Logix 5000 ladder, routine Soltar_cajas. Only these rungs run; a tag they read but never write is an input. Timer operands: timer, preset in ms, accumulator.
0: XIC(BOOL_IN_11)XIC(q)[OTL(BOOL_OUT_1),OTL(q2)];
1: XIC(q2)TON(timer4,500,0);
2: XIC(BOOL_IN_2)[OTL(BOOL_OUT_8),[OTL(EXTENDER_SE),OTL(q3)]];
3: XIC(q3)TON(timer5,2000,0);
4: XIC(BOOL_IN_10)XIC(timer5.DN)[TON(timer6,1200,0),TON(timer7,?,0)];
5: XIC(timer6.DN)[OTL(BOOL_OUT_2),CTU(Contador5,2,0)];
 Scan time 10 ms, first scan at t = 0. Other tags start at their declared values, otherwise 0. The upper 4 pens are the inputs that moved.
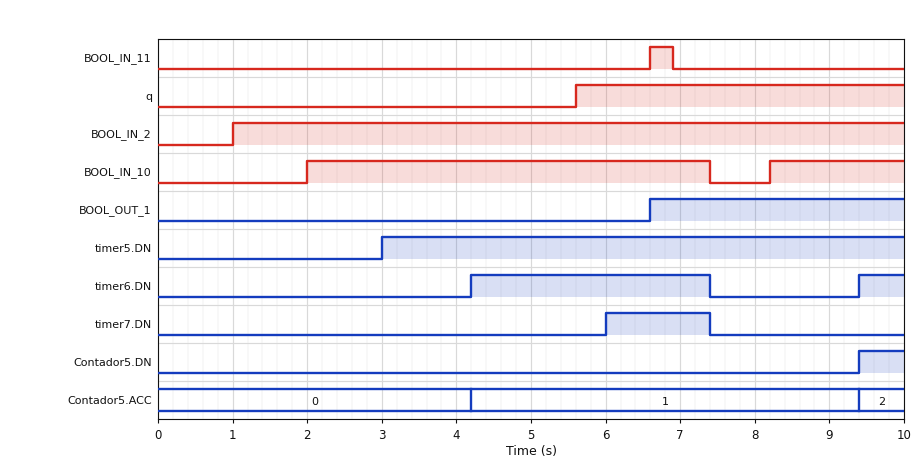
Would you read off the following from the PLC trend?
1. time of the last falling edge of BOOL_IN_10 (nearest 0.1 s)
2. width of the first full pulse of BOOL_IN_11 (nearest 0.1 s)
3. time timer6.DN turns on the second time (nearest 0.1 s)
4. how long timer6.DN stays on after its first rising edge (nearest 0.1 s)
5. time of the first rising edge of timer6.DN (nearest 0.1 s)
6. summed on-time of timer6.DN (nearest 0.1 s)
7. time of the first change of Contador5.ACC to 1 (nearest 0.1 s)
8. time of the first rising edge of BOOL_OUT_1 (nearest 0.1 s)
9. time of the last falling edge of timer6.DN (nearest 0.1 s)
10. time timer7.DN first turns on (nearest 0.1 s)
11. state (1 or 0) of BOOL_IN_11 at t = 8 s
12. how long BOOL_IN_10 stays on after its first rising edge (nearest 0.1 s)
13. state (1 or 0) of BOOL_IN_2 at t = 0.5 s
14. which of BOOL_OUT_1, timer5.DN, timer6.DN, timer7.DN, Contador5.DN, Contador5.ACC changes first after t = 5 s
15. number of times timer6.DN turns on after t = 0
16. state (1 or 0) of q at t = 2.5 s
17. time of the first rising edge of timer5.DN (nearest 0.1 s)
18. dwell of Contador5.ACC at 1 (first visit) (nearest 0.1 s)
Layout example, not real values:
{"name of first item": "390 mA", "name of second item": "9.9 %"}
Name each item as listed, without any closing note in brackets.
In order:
{"time of the last falling edge of BOOL_IN_10": "7.4 s", "width of the first full pulse of BOOL_IN_11": "0.3 s", "time timer6.DN turns on the second time": "9.4 s", "how long timer6.DN stays on after its first rising edge": "3.2 s", "time of the first rising edge of timer6.DN": "4.2 s", "summed on-time of timer6.DN": "3.8 s", "time of the first change of Contador5.ACC to 1": "4.2 s", "time of the first rising edge of BOOL_OUT_1": "6.6 s", "time of the last falling edge of timer6.DN": "7.4 s", "time timer7.DN first turns on": "6.0 s", "state (1 or 0) of BOOL_IN_11 at t = 8 s": "0", "how long BOOL_IN_10 stays on after its first rising edge": "5.4 s", "state (1 or 0) of BOOL_IN_2 at t = 0.5 s": "0", "which of BOOL_OUT_1, timer5.DN, timer6.DN, timer7.DN, Contador5.DN, Contador5.ACC changes first after t = 5 s": "timer7.DN", "number of times timer6.DN turns on after t = 0": "2", "state (1 or 0) of q at t = 2.5 s": "0", "time of the first rising edge of timer5.DN": "3.0 s", "dwell of Contador5.ACC at 1 (first visit)": "5.2 s"}
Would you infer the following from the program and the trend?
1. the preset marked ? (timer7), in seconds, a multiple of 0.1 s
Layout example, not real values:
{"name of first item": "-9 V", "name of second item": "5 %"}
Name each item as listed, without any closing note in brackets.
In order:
{"the preset marked ? (timer7), in seconds, a multiple of 0.1 s": "3.0 s"}
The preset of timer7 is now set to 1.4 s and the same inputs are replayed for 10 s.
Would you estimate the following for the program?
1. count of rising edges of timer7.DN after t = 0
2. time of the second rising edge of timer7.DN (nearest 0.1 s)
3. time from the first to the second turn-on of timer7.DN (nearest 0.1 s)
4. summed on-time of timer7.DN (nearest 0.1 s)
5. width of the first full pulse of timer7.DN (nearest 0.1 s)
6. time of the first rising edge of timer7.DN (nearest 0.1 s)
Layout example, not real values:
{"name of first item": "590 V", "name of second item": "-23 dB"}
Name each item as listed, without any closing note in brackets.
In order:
{"count of rising edges of timer7.DN after t = 0": "2", "time of the second rising edge of timer7.DN": "9.6 s", "time from the first to the second turn-on of timer7.DN": "5.2 s", "summed on-time of timer7.DN": "3.4 s", "width of the first full pulse of timer7.DN": "3.0 s", "time of the first rising edge of timer7.DN": "4.4 s"}
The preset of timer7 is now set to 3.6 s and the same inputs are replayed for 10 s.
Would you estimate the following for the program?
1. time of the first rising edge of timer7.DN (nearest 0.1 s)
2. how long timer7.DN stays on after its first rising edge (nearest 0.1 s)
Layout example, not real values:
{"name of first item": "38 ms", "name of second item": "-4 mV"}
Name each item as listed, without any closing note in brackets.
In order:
{"time of the first rising edge of timer7.DN": "6.6 s", "how long timer7.DN stays on after its first rising edge": "0.8 s"}
